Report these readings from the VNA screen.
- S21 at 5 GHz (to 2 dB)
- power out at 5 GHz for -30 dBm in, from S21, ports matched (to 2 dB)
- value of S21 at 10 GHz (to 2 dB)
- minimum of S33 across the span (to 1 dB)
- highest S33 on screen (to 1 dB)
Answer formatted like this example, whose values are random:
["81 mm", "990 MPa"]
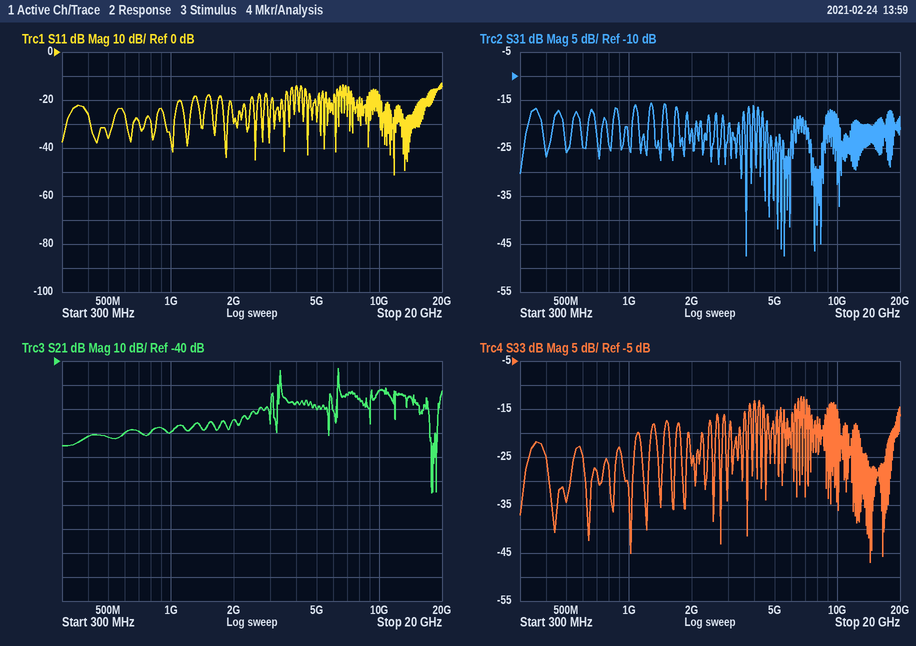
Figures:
["-60 dB", "-90 dBm", "-52 dB", "-47 dB", "-12 dB"]
